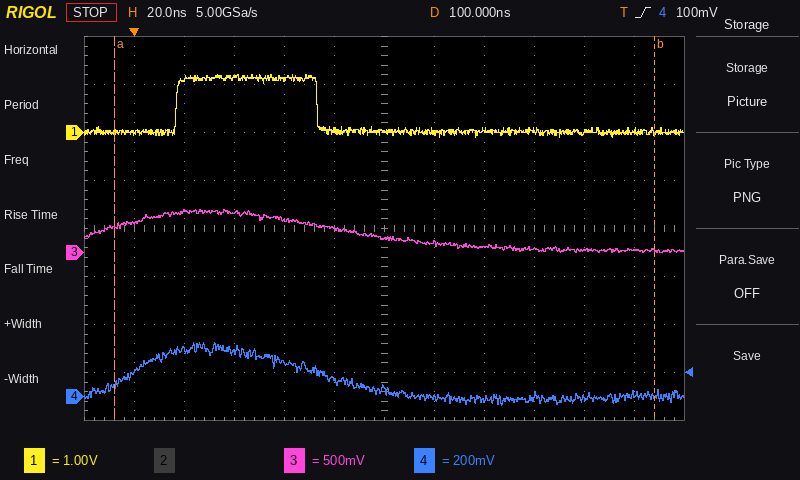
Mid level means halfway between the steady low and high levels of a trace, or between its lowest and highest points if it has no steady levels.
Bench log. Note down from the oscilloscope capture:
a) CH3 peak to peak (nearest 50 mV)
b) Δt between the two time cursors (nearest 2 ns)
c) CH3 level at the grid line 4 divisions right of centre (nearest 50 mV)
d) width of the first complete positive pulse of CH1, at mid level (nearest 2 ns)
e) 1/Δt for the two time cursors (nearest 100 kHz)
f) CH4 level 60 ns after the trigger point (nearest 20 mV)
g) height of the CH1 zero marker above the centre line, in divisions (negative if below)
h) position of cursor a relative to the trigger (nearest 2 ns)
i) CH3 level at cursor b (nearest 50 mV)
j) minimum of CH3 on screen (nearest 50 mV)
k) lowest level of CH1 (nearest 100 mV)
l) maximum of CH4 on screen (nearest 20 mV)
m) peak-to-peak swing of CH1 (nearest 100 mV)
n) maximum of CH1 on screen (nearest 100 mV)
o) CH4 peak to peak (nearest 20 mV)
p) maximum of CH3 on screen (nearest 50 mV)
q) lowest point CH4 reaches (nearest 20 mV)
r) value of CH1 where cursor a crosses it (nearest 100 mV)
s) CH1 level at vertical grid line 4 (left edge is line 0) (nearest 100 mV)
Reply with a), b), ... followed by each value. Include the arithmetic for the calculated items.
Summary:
a) 450 mV − (0 mV) = 450 mV
b) 216 ns
c) 50 mV
d) 56 ns
e) 1 / 216 ns ≈ 4.6 MHz
f) 140 mV
g) +2.0 div
h) -8 ns
i) 0 mV
j) 0 mV
k) -100 mV
l) 220 mV
m) 1.2 V − (-100 mV) = 1.3 V
n) 1.2 V
o) 220 mV − (-40 mV) = 260 mV
p) 450 mV
q) -40 mV
r) 0.0 V
s) 1.1 V
